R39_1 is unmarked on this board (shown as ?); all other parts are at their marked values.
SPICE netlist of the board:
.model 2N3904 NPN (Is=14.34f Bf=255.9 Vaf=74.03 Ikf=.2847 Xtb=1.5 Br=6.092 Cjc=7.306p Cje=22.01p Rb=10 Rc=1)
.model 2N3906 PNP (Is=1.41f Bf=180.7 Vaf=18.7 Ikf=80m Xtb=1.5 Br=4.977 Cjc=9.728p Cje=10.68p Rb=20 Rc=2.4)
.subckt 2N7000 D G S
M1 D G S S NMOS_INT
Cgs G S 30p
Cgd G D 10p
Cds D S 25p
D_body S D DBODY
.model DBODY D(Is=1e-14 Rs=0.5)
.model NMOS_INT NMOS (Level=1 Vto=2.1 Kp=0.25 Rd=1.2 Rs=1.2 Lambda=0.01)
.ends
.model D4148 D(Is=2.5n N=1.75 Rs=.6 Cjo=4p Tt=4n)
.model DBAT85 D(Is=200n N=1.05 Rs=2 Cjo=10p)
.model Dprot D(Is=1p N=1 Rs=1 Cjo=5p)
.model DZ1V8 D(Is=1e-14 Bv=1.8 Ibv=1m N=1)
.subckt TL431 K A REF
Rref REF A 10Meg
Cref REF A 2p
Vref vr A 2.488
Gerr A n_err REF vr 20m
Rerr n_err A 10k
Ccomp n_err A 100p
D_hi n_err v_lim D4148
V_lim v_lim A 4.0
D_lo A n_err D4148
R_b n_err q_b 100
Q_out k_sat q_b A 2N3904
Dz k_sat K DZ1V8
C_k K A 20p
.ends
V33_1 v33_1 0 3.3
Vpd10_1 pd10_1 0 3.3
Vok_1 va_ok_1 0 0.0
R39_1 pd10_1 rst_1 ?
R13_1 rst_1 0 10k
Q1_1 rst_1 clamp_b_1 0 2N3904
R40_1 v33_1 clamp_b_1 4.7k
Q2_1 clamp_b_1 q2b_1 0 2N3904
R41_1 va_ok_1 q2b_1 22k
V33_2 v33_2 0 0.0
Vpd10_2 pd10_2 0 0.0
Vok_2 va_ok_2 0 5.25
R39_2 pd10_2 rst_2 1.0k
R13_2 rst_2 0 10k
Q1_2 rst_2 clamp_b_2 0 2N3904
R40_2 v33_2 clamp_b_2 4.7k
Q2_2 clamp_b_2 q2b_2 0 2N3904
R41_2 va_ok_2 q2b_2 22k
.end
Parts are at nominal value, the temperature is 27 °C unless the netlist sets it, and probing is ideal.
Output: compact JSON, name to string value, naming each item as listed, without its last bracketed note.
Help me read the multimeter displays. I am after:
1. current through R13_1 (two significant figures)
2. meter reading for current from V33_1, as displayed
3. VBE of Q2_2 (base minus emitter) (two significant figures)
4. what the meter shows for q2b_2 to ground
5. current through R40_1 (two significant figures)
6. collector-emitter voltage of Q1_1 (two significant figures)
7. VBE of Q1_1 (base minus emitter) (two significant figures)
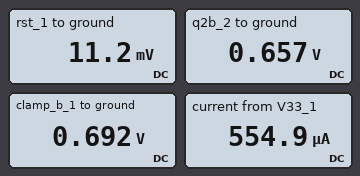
{"current through R13_1": "1.1 µA", "meter reading for current from V33_1, as displayed": "554.9 µA", "VBE of Q2_2 (base minus emitter)": "660 mV", "what the meter shows for q2b_2 to ground": "0.657 V", "current through R40_1": "550 µA", "collector-emitter voltage of Q1_1": "11 mV", "VBE of Q1_1 (base minus emitter)": "690 mV"}
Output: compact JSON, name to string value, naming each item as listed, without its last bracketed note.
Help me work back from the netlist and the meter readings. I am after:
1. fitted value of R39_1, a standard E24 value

{"fitted value of R39_1, a standard E24 value": "3.3 kΩ"}
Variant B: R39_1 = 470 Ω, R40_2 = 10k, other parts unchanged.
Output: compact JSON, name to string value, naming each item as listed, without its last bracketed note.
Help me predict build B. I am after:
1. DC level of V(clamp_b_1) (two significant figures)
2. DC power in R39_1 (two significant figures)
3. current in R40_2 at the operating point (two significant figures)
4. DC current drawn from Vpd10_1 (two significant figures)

{"DC level of V(clamp_b_1)": "710 mV", "DC power in R39_1": "23 mW", "current in R40_2 at the operating point": "400 nA", "DC current drawn from Vpd10_1": "6.9 mA"}
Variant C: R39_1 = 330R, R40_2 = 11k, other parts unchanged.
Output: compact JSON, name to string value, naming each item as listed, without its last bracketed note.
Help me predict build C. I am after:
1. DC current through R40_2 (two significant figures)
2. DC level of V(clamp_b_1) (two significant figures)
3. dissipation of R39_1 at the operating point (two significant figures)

{"DC current through R40_2": "360 nA", "DC level of V(clamp_b_1)": "720 mV", "dissipation of R39_1 at the operating point": "32 mW"}
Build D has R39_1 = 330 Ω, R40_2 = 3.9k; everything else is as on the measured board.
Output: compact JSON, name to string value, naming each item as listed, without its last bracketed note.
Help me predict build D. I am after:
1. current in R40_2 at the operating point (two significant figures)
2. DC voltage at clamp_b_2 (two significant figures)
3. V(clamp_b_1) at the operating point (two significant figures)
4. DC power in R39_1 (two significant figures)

{"current in R40_2 at the operating point": "1.0 µA", "DC voltage at clamp_b_2": "4.0 mV", "V(clamp_b_1) at the operating point": "720 mV", "DC power in R39_1": "32 mW"}
